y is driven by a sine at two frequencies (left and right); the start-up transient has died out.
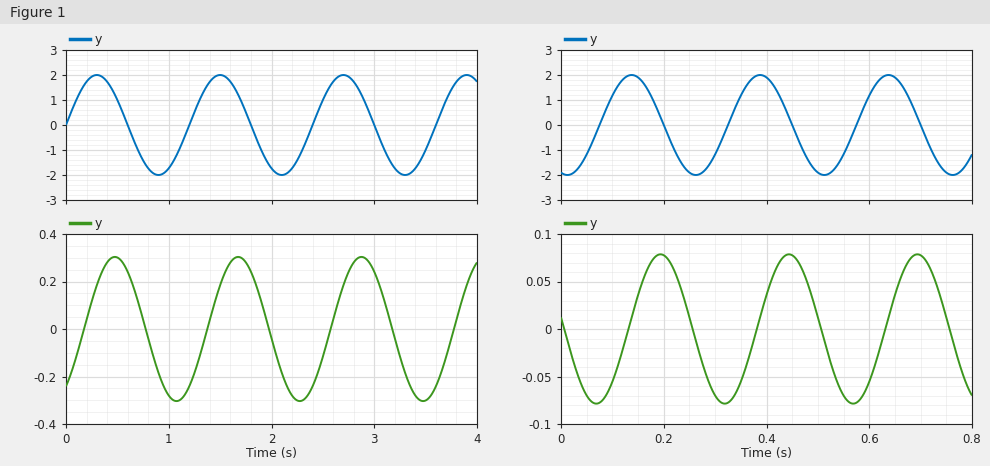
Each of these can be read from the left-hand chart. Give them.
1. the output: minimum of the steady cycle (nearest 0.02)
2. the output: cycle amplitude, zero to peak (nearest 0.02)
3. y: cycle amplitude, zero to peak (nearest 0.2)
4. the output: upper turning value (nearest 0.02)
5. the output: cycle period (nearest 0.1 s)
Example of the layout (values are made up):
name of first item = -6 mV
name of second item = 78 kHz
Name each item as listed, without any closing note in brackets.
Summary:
the output: minimum of the steady cycle = -0.30
the output: cycle amplitude, zero to peak = 0.30
y: cycle amplitude, zero to peak = 2.0
the output: upper turning value = 0.30
the output: cycle period = 1.2 s
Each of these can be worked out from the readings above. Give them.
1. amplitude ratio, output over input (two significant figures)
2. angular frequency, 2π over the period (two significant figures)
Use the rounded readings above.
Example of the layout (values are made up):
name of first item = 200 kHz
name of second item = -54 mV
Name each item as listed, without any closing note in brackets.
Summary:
amplitude ratio, output over input = 0.15
angular frequency, 2π over the period = 5.2 rad/s
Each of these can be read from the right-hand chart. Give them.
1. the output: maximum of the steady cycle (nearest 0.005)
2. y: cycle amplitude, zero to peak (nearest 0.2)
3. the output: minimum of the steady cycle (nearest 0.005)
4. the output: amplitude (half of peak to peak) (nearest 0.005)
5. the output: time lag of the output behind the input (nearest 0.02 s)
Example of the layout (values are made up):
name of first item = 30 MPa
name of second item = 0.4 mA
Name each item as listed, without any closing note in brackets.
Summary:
the output: maximum of the steady cycle = 0.080
y: cycle amplitude, zero to peak = 2.0
the output: minimum of the steady cycle = -0.080
the output: amplitude (half of peak to peak) = 0.080
the output: time lag of the output behind the input = 0.06 s
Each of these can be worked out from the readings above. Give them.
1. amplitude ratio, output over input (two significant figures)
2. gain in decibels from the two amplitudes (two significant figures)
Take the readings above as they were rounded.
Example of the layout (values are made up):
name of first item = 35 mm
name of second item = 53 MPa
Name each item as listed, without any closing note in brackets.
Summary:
amplitude ratio, output over input = 0.040
gain in decibels from the two amplitudes = -28 dB
